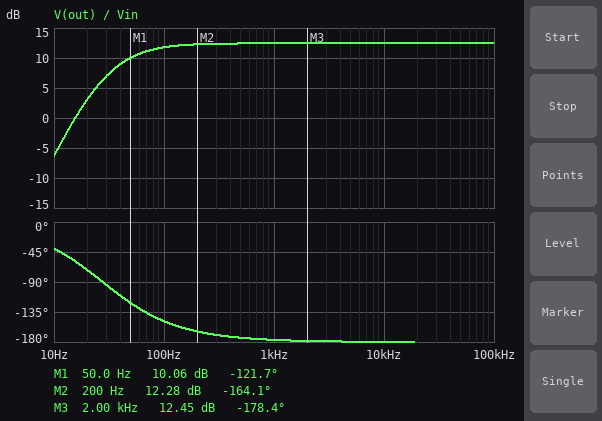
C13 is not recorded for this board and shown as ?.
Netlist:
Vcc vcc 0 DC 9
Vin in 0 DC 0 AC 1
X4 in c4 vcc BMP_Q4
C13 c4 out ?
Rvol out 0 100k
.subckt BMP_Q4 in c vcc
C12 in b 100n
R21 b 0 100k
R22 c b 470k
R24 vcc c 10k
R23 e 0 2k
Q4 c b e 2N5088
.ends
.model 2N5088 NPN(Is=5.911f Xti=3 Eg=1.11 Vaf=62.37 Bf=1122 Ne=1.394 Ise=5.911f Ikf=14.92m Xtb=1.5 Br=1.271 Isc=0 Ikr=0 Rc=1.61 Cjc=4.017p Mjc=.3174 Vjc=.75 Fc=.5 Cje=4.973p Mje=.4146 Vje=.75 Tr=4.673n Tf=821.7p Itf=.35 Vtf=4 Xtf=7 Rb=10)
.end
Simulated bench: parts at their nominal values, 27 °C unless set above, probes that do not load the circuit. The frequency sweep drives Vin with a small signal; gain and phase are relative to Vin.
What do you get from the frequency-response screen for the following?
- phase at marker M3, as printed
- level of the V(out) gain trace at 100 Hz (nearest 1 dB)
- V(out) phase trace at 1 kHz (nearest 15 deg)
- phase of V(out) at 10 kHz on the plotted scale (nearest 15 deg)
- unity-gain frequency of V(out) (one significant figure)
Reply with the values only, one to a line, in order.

-178.4 deg
12 dB
-180 deg
-180 deg
20 Hz
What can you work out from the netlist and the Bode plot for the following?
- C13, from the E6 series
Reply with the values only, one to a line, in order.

68 nF
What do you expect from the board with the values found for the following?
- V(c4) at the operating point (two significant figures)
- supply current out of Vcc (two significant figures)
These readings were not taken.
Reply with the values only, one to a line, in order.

6.5 V
250 µA
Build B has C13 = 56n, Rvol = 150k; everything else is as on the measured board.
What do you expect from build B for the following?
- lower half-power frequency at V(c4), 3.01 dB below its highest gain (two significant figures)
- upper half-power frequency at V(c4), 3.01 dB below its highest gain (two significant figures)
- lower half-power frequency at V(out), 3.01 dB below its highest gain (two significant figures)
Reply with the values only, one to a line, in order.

34 Hz
9.2 MHz
42 Hz
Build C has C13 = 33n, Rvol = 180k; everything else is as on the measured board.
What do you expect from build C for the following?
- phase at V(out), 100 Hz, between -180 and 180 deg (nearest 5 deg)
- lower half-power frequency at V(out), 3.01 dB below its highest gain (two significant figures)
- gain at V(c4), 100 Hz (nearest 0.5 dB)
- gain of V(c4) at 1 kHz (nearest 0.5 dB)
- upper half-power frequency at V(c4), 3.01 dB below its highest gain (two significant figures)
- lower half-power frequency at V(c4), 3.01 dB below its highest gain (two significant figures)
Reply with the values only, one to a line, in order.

-145 deg
47 Hz
12.5 dB
13.0 dB
9.1 MHz
34 Hz
